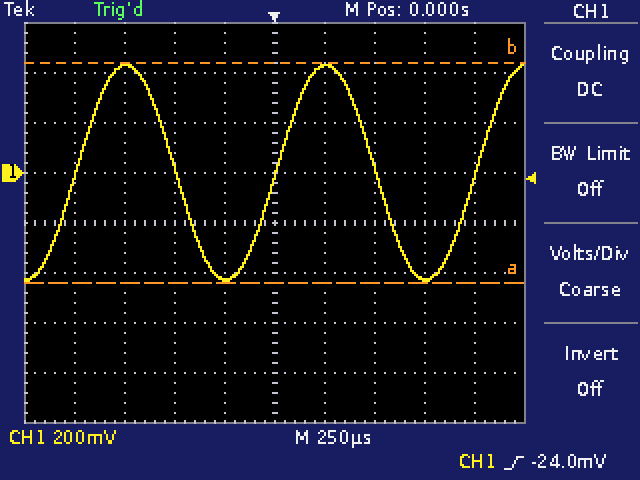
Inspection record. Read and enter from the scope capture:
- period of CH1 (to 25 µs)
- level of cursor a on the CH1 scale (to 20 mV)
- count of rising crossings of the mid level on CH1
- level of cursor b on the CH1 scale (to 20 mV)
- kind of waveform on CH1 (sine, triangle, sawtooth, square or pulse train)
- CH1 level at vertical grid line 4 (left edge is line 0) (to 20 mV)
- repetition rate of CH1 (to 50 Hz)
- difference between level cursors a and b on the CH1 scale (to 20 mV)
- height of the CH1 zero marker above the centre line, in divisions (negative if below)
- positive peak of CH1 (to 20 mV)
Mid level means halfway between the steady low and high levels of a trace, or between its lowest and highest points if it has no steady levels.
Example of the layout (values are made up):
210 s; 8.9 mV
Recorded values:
1.000 ms; -440 mV; 3; 440 mV; sine; -420 mV; 1.00 kHz; 880 mV; +1.0 div; 440 mV
